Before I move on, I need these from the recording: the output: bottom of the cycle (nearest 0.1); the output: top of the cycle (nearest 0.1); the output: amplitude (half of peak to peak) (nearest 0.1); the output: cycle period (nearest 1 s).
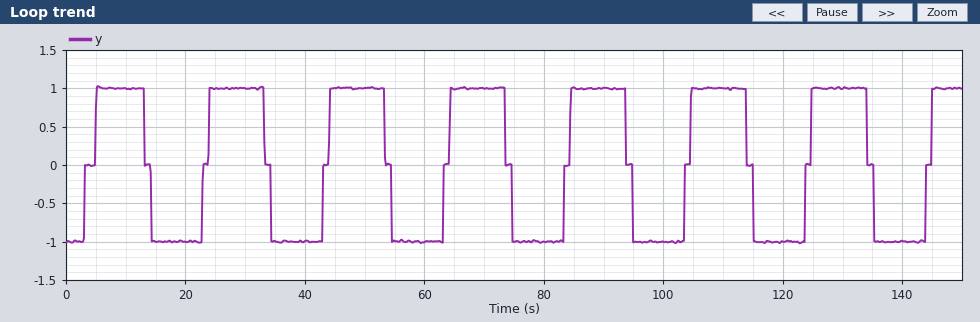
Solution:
-1.0
1.0
1.0
20 s
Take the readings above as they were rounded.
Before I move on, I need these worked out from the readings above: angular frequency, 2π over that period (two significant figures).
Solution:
0.31 rad/s
